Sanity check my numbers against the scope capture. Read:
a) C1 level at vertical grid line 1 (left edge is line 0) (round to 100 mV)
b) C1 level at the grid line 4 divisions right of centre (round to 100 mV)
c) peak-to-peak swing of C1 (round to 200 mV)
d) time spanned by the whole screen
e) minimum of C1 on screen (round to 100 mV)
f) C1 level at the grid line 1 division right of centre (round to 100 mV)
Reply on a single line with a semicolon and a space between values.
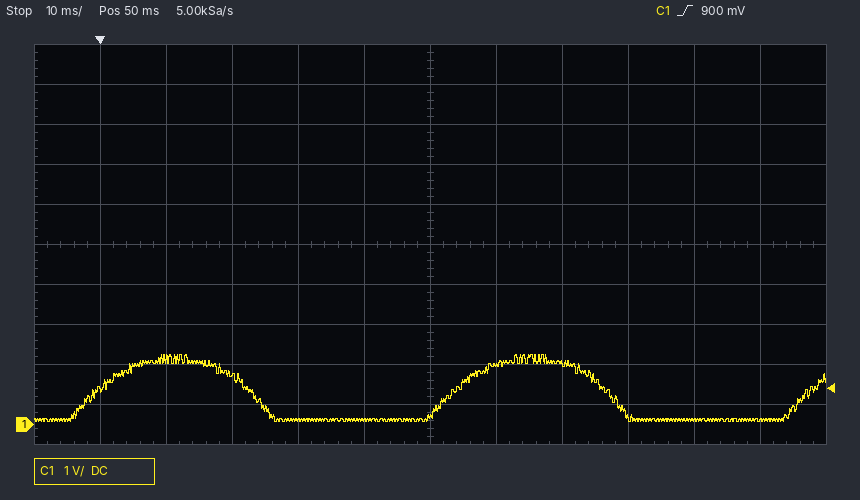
900 mV; 100 mV; 1.6 V; 120 ms; 100 mV; 1.5 V
